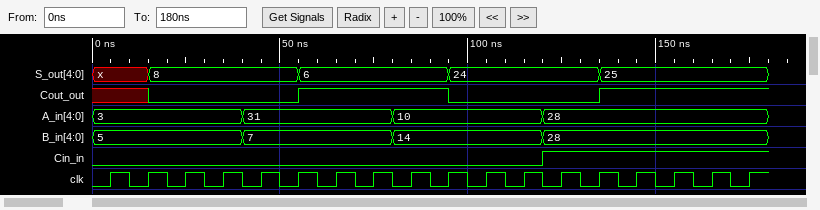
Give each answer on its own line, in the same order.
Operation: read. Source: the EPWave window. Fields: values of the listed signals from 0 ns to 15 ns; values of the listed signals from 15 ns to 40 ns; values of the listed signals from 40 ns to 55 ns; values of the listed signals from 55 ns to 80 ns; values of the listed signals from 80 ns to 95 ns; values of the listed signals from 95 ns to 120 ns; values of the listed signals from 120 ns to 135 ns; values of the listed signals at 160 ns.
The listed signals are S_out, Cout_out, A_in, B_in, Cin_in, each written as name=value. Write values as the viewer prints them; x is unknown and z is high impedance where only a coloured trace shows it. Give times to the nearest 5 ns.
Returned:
S_out=x, Cout_out=x, A_in=3, B_in=5, Cin_in=0
S_out=8, Cout_out=0, A_in=3, B_in=5, Cin_in=0
S_out=8, Cout_out=0, A_in=31, B_in=7, Cin_in=0
S_out=6, Cout_out=1, A_in=31, B_in=7, Cin_in=0
S_out=6, Cout_out=1, A_in=10, B_in=14, Cin_in=0
S_out=24, Cout_out=0, A_in=10, B_in=14, Cin_in=0
S_out=24, Cout_out=0, A_in=28, B_in=28, Cin_in=1
S_out=25, Cout_out=1, A_in=28, B_in=28, Cin_in=1
